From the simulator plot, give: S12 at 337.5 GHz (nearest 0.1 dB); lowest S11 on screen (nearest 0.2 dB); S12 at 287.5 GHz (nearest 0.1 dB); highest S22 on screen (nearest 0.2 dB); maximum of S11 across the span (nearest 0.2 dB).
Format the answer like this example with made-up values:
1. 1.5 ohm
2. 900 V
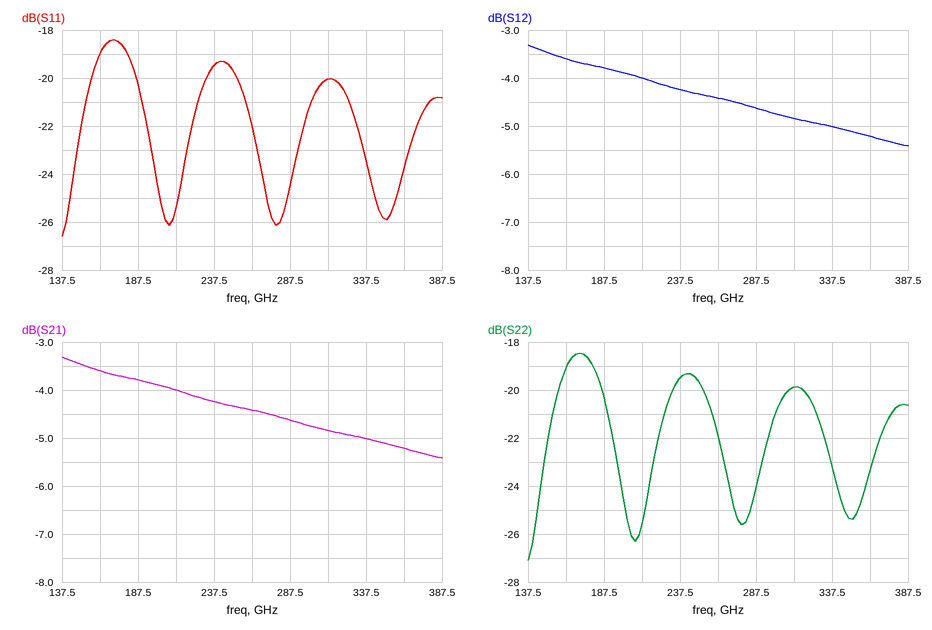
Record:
1. -5.0 dB
2. -26.6 dB
3. -4.6 dB
4. -18.4 dB
5. -18.4 dB
